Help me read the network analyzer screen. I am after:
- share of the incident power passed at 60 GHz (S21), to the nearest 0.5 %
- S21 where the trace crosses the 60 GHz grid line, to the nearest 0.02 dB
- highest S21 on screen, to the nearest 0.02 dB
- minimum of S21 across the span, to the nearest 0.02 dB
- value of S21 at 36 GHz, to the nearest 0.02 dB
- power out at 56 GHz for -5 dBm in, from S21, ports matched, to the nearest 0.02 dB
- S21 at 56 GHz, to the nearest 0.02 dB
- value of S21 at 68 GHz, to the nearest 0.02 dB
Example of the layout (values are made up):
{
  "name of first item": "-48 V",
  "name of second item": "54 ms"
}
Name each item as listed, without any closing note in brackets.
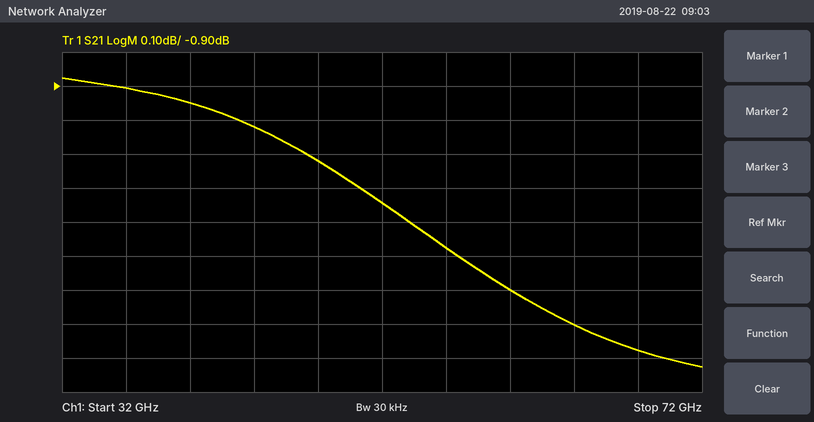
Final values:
{
  "share of the incident power passed at 60 GHz (S21), to the nearest 0.5 %": "71.0 %",
  "S21 where the trace crosses the 60 GHz grid line, to the nearest 0.02 dB": "-1.50 dB",
  "highest S21 on screen, to the nearest 0.02 dB": "-0.88 dB",
  "minimum of S21 across the span, to the nearest 0.02 dB": "-1.72 dB",
  "value of S21 at 36 GHz, to the nearest 0.02 dB": "-0.90 dB",
  "power out at 56 GHz for -5 dBm in, from S21, ports matched, to the nearest 0.02 dB": "-6.38 dBm",
  "S21 at 56 GHz, to the nearest 0.02 dB": "-1.38 dB",
  "value of S21 at 68 GHz, to the nearest 0.02 dB": "-1.68 dB"
}
